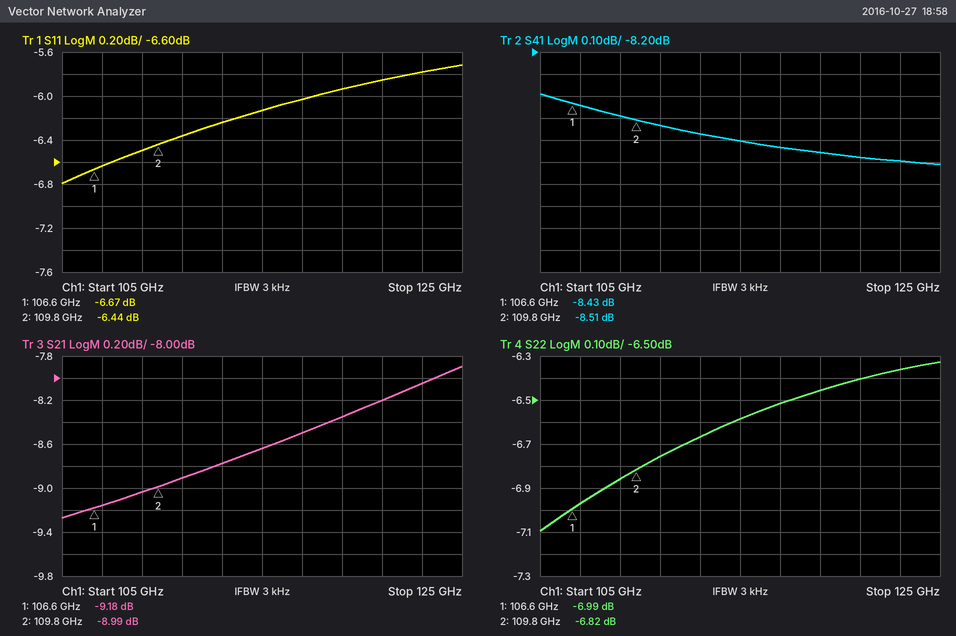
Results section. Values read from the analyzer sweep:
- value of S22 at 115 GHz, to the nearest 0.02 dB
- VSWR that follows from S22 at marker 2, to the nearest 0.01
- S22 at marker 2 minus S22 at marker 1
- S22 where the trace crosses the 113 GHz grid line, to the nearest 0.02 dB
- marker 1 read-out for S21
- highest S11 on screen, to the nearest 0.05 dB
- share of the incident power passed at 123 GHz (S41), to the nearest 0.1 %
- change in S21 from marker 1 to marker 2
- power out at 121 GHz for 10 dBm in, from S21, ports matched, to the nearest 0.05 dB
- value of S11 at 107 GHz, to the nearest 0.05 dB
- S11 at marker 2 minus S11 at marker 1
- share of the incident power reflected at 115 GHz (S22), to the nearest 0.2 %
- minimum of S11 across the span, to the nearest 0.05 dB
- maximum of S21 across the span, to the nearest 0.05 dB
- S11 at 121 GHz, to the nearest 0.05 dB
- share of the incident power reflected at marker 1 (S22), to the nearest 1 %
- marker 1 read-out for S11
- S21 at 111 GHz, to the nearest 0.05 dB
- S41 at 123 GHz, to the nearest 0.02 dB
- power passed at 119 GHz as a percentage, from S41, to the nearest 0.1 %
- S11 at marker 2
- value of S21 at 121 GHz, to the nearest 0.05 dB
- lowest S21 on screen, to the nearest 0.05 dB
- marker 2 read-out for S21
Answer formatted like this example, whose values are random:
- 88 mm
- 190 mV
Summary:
- -6.58 dB
- 2.68
- 0.17 dB
- -6.66 dB
- -9.18 dB
- -5.70 dB
- 13.5 %
- 0.19 dB
- 1.80 dBm
- -6.65 dB
- 0.23 dB
- 22.0 %
- -6.80 dB
- -7.90 dB
- -5.85 dB
- 20 %
- -6.67 dB
- -8.90 dB
- -8.70 dB
- 13.6 %
- -6.44 dB
- -8.20 dB
- -9.25 dB
- -8.99 dB
